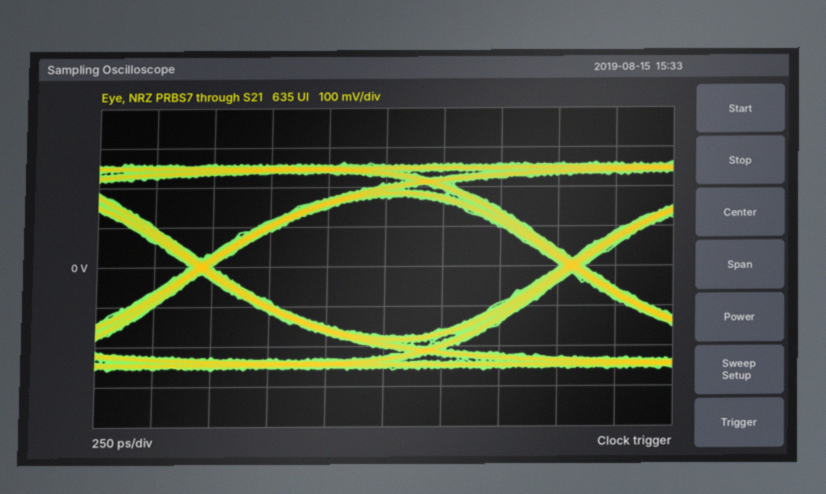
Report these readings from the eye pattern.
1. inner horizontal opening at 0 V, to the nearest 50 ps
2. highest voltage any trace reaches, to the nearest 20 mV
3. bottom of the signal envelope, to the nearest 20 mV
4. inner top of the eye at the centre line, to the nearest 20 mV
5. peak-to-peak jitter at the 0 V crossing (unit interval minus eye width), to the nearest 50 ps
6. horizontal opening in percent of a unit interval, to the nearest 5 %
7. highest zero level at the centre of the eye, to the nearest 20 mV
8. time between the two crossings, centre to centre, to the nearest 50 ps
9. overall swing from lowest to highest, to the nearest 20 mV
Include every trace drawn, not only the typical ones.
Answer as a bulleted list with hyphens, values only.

- 1.50 ns
- 260 mV
- -260 mV
- 180 mV
- 100 ps
- 95 %
- -180 mV
- 1.60 ns
- 520 mV
